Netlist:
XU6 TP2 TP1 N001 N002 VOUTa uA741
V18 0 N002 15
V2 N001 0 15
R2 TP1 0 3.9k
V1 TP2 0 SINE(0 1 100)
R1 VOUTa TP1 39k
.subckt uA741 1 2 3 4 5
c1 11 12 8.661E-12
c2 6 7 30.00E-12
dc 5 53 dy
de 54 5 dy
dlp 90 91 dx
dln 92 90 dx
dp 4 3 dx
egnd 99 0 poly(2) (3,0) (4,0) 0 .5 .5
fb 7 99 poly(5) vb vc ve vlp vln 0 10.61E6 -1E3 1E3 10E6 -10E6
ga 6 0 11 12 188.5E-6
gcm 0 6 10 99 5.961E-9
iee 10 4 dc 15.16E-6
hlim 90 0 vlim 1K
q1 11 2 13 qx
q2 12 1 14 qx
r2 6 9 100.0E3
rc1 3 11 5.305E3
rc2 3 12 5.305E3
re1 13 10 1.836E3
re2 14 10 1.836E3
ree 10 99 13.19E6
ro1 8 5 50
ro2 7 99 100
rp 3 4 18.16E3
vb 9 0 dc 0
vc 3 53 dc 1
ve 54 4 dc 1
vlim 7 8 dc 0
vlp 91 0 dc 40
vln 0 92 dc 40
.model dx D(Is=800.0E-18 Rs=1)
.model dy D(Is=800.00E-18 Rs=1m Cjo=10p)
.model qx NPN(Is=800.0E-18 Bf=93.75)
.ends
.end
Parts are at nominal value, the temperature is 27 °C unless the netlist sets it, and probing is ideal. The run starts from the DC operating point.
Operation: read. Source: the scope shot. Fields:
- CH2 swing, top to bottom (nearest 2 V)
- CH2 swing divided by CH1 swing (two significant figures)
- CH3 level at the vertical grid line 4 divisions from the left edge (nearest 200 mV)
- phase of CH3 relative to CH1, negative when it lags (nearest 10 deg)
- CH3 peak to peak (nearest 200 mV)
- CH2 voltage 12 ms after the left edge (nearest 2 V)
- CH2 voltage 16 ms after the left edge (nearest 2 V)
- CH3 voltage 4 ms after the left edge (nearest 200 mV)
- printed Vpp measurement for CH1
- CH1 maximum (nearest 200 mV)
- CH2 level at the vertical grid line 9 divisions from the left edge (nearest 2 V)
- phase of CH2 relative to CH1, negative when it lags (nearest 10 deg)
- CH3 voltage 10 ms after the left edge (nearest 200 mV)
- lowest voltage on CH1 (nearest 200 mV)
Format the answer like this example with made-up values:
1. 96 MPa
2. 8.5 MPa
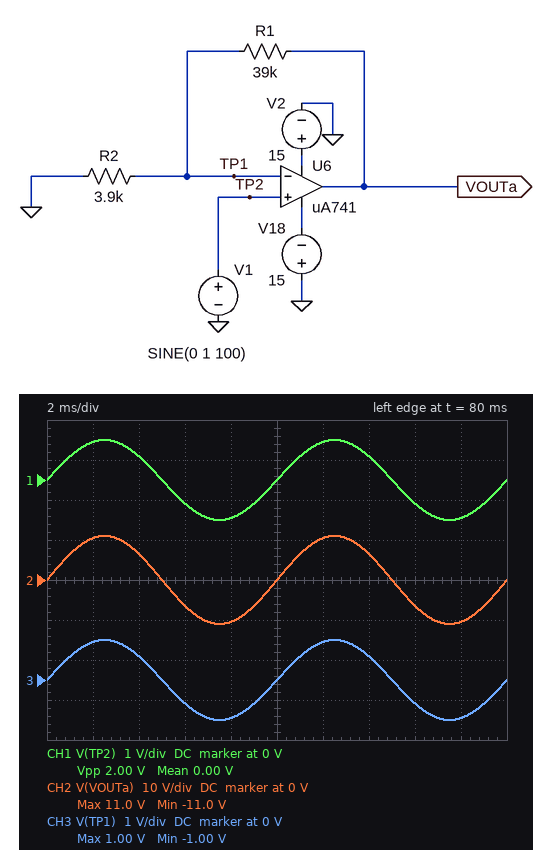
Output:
1. 22 V
2. 11
3. -1.0 V
4. 0 deg
5. 2.0 V
6. 10 V
7. -6 V
8. 600 mV
9. 2.00 V
10. 1.0 V
11. -10 V
12. 0 deg
13. 0 V
14. -1.0 V
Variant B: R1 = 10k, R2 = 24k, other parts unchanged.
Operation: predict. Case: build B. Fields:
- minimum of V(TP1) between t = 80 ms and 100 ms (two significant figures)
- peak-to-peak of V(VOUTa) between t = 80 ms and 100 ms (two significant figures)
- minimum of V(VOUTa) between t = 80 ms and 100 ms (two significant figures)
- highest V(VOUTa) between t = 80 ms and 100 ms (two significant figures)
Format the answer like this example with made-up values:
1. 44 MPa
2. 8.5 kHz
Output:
1. -1.0 V
2. 2.8 V
3. -1.4 V
4. 1.4 V
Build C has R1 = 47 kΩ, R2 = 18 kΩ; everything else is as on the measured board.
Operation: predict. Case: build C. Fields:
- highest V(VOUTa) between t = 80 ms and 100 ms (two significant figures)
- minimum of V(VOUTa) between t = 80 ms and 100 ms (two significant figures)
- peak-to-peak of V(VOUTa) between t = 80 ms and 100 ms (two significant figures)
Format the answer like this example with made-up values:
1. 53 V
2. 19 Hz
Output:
1. 3.6 V
2. -3.6 V
3. 7.2 V
